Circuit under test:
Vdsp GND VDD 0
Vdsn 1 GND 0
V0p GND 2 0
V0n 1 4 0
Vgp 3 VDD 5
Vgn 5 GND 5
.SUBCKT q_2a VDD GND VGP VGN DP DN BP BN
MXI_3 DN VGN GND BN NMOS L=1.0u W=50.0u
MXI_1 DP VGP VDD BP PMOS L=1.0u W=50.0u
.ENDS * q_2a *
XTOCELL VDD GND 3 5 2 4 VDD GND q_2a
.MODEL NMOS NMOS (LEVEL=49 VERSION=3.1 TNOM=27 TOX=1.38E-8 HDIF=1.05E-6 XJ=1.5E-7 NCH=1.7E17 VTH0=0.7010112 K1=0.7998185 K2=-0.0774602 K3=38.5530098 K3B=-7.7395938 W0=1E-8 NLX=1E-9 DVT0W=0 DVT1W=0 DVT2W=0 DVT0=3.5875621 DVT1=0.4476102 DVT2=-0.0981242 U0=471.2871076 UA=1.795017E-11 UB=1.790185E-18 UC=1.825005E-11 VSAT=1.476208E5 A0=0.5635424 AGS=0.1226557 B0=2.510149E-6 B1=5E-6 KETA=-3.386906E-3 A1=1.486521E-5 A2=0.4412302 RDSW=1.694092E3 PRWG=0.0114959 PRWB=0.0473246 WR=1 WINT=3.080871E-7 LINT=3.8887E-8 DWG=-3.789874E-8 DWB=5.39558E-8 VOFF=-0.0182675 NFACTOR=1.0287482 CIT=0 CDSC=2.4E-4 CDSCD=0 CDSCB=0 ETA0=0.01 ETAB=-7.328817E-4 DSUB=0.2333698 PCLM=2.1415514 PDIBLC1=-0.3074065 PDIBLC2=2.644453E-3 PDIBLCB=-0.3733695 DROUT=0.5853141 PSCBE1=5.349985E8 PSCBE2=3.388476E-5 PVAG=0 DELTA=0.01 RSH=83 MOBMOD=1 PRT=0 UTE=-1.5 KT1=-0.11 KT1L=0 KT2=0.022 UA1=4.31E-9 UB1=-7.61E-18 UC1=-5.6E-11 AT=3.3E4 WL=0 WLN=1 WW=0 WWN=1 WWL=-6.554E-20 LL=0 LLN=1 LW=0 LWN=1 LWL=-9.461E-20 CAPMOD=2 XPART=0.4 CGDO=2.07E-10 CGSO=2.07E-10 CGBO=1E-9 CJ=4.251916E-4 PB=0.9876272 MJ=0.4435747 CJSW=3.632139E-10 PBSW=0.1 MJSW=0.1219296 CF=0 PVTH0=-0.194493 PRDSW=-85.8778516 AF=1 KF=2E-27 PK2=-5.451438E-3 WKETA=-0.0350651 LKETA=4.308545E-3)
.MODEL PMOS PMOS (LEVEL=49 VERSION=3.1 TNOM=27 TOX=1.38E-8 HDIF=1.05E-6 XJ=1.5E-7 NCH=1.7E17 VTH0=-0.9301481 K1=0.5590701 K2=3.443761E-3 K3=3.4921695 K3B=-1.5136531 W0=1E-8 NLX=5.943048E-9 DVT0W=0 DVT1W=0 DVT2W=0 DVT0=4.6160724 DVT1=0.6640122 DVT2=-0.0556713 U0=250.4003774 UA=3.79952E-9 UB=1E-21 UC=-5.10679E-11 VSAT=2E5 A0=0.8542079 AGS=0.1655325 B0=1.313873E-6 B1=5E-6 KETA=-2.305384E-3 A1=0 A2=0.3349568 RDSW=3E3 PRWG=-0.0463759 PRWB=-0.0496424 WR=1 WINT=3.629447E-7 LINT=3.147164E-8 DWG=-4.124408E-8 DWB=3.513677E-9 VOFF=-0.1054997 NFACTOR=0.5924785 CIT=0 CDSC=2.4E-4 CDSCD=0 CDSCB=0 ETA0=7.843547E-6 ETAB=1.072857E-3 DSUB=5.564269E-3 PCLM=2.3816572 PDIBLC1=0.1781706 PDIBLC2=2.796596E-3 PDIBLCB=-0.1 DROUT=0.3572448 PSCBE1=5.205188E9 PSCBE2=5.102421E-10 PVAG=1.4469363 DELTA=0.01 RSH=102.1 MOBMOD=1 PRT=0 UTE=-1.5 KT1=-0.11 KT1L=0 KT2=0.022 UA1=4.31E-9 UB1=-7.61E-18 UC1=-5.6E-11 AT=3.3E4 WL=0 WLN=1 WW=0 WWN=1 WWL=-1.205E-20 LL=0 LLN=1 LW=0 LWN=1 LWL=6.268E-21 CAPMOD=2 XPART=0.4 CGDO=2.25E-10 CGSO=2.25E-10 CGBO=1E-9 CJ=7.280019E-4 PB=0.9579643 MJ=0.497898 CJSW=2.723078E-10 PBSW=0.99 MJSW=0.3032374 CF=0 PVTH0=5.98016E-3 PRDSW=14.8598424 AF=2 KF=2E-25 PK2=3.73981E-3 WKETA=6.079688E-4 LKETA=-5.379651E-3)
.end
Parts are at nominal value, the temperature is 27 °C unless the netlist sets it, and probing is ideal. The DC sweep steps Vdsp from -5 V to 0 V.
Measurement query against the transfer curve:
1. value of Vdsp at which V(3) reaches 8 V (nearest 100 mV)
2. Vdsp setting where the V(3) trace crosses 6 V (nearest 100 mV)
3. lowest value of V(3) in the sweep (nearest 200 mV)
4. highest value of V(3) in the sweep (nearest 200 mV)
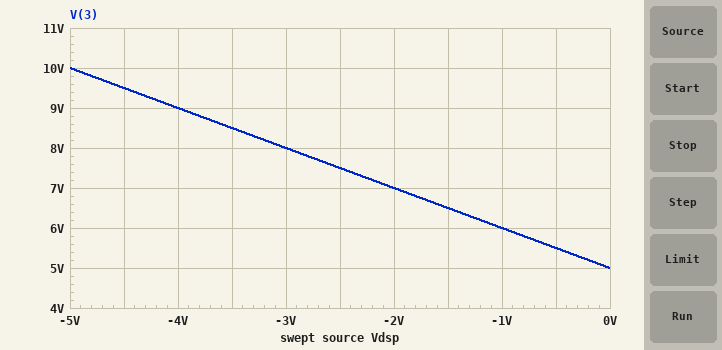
-3.0 V
-1.0 V
5.0 V
10.0 V
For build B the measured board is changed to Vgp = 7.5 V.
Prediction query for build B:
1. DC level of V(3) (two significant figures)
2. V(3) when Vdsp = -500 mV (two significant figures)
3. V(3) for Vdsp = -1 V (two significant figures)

7.5 V
8.0 V
8.5 V
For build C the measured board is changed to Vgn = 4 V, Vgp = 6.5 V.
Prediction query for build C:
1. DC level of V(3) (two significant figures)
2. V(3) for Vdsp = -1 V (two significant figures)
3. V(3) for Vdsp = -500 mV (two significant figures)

6.5 V
7.5 V
7.0 V
